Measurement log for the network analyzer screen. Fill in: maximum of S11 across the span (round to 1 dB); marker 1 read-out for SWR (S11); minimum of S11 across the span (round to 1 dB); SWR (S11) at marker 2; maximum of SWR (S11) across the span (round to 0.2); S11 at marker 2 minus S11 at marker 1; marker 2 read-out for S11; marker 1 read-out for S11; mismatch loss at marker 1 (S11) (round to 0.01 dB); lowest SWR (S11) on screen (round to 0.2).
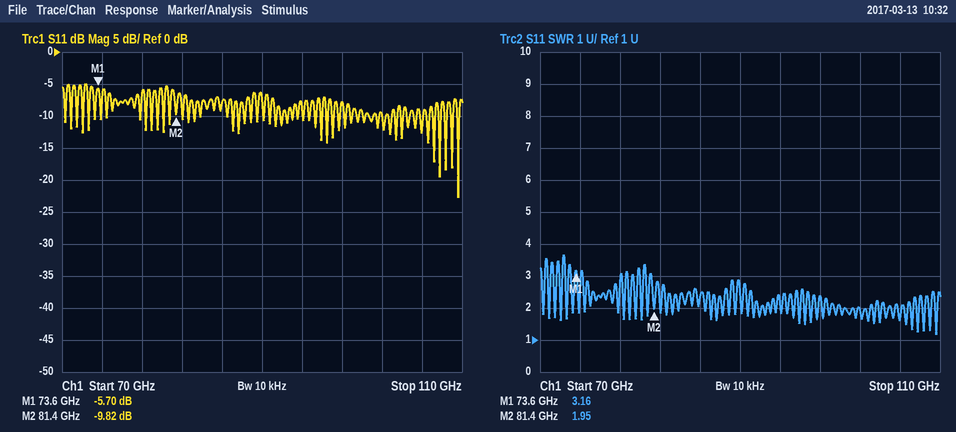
-5 dB
3.16
-23 dB
1.95
3.6
-4.12 dB
-9.82 dB
-5.70 dB
1.36 dB
1.2
